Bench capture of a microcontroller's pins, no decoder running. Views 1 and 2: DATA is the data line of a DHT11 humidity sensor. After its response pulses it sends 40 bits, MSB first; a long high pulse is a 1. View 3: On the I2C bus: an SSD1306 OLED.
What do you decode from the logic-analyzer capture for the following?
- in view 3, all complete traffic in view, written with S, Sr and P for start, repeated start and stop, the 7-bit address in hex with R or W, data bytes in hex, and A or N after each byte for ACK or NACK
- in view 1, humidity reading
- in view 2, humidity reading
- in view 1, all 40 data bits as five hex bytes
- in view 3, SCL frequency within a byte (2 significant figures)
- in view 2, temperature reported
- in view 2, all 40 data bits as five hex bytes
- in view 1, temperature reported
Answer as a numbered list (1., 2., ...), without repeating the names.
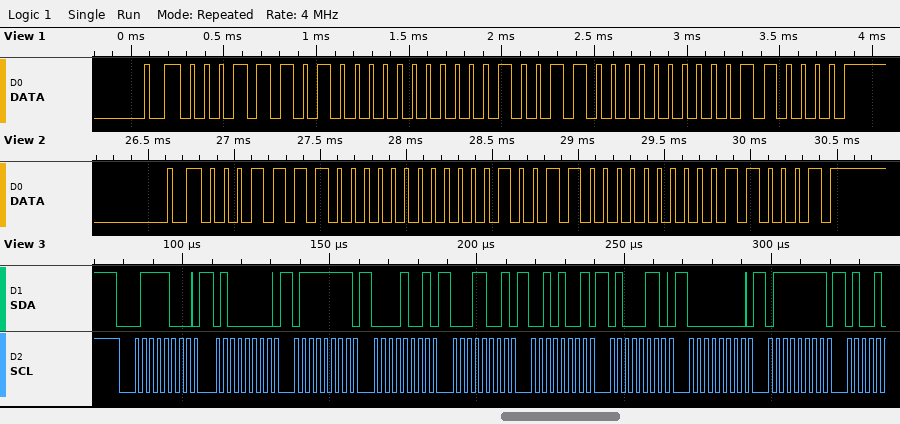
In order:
1. S 3CW A 40 A 7F A 09 A 19 A 29 A 46 A 00 A 7F A
2. 29 %
3. 30 %
4. 1D 00 13 00 30
5. 400 kHz
6. 19.0 °C
7. 1E 00 13 00 31
8. 19.0 °C
